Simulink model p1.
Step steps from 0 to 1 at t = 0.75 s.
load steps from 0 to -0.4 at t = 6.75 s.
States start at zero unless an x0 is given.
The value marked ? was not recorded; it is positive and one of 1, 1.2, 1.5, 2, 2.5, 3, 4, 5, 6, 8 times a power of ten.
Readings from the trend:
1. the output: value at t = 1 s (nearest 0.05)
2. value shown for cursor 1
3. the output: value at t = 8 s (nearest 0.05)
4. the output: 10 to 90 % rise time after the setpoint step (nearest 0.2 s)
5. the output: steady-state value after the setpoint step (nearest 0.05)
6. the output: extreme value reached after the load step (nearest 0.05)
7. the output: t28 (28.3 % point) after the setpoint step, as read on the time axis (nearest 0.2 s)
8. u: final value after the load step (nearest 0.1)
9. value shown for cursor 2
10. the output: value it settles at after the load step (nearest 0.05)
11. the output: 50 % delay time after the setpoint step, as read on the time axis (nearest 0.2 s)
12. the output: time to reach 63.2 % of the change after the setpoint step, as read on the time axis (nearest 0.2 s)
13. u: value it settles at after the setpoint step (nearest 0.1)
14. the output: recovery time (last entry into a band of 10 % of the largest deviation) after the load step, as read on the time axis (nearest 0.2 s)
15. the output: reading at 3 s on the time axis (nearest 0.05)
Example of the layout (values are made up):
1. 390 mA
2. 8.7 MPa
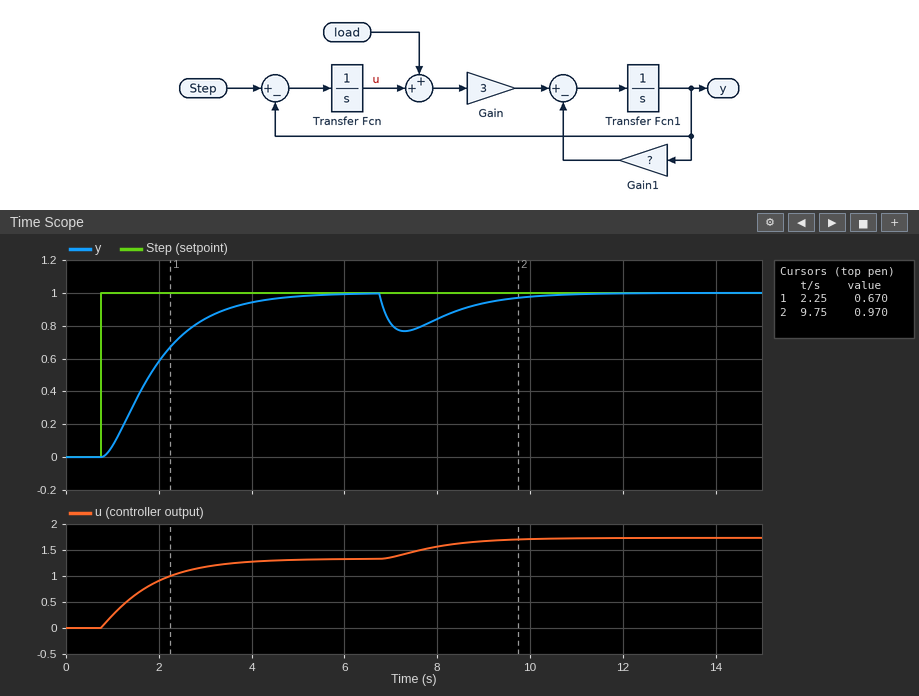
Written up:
1. 0.05
2. 0.670
3. 0.85
4. 2.4 s
5. 1.00
6. 0.75
7. 1.4 s
8. 1.7
9. 0.970
10. 1.00
11. 1.8 s
12. 2.2 s
13. 1.3
14. 10.0 s
15. 0.85
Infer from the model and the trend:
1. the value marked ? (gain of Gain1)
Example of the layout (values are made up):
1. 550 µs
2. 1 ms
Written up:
1. 4
